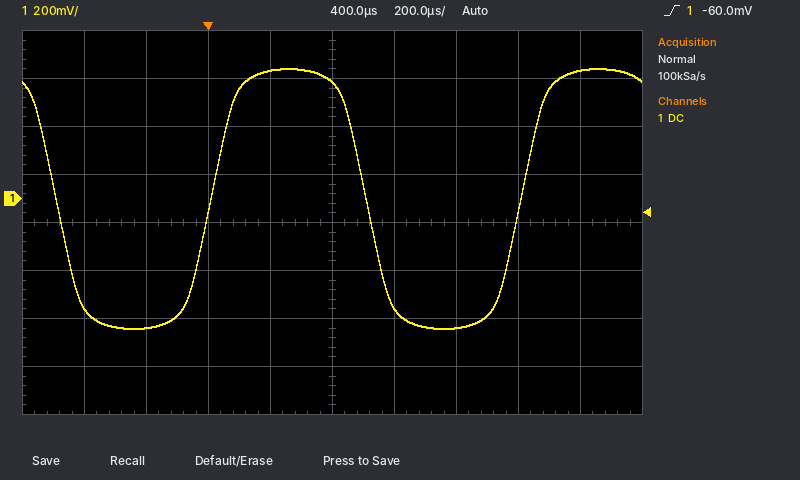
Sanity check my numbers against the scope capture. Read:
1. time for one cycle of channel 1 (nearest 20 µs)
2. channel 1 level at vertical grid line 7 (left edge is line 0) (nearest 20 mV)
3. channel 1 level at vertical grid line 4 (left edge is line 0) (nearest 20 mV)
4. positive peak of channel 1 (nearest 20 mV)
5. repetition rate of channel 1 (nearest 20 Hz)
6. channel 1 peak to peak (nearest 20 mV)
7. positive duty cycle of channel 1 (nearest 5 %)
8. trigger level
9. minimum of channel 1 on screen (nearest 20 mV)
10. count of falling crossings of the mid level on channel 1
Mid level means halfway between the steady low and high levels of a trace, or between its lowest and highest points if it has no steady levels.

1.00 ms
-540 mV
540 mV
540 mV
1.00 kHz
1.08 V
50 %
-60.0 mV
-540 mV
2
